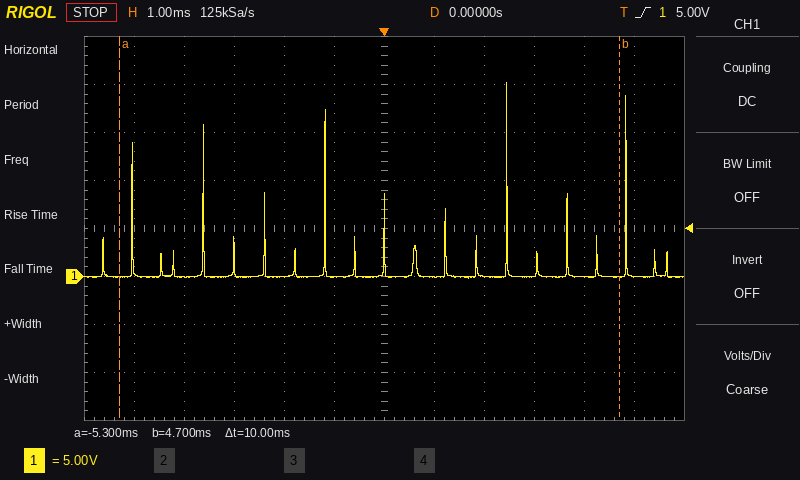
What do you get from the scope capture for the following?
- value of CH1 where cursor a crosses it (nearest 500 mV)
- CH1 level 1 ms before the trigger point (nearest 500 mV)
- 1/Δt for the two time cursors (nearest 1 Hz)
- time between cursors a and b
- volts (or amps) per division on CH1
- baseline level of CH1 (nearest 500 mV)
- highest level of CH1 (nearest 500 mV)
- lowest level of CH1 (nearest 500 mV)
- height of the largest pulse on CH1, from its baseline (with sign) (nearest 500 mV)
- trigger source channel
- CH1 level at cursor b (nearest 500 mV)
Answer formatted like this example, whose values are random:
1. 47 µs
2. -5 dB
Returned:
1. 0.0 V
2. 0.0 V
3. 100 Hz
4. 10 ms
5. 5 V
6. 0.0 V
7. 20.0 V
8. 0.0 V
9. +20.0 V
10. CH1
11. 0.0 V
